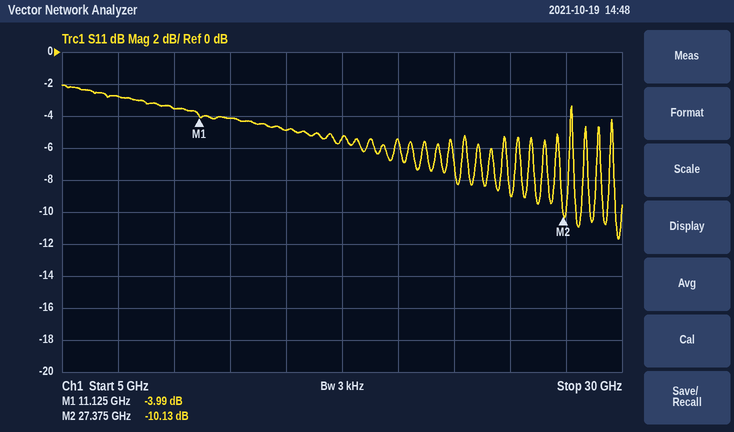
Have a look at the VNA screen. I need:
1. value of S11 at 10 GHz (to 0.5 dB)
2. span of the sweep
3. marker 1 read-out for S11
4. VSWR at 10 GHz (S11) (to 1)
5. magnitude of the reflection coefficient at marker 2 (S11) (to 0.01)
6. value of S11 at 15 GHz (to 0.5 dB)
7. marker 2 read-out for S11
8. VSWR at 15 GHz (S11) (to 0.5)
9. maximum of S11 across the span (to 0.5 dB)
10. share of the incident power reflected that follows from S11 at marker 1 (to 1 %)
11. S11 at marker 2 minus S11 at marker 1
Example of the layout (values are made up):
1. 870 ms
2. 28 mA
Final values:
1. -3.5 dB
2. 25 GHz
3. -3.99 dB
4. 5
5. 0.31
6. -5.0 dB
7. -10.13 dB
8. 3.5
9. -2.0 dB
10. 40 %
11. -6.14 dB
